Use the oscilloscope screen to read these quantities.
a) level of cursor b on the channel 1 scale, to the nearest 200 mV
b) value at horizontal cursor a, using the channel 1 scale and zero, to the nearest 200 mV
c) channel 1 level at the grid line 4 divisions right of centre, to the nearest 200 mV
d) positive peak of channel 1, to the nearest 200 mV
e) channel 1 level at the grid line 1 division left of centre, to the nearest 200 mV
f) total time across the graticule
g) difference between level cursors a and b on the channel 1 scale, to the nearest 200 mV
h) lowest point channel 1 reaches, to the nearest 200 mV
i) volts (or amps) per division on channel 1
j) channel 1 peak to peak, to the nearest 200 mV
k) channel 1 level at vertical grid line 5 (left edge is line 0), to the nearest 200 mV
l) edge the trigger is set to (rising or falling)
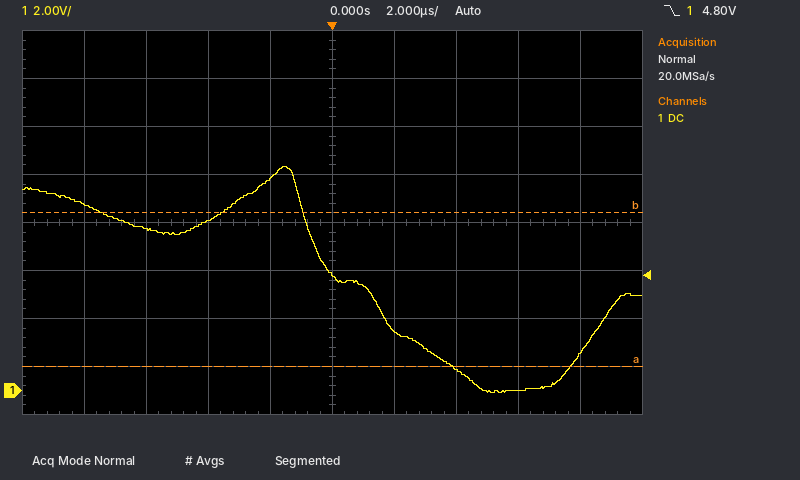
7.4 V
1.0 V
1.6 V
9.4 V
8.8 V
20 µs
6.4 V
0.0 V
2 V
9.4 V
4.8 V
falling
